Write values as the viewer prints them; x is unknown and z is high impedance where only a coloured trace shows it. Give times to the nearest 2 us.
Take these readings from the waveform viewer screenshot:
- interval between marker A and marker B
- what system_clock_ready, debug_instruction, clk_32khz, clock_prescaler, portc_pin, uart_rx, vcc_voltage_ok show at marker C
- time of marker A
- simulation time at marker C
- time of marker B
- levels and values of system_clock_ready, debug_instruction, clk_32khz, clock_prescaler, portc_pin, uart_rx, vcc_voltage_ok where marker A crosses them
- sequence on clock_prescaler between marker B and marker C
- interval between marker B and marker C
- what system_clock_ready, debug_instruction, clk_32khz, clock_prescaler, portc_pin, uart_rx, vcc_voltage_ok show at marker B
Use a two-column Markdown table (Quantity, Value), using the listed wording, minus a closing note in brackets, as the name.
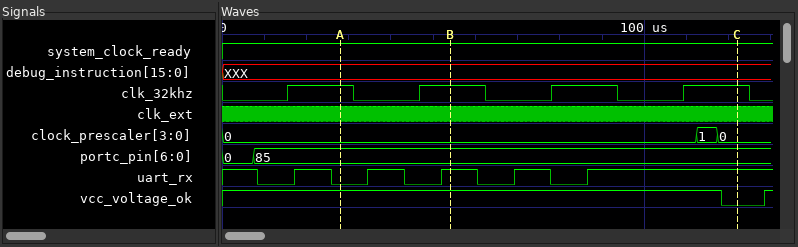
| Quantity | Value |
|---|---|
| interval between marker A and marker B | 26 us |
| what system_clock_ready, debug_instruction, clk_32khz, clock_prescaler, portc_pin, uart_rx, vcc_voltage_ok show at marker C | system_clock_ready=1, debug_instruction=XXX, clk_32khz=1, clock_prescaler=0, portc_pin=85, uart_rx=1, vcc_voltage_ok=0 |
| time of marker A | 28 us |
| simulation time at marker C | 122 us |
| time of marker B | 54 us |
| levels and values of system_clock_ready, debug_instruction, clk_32khz, clock_prescaler, portc_pin, uart_rx, vcc_voltage_ok where marker A crosses them | system_clock_ready=1, debug_instruction=XXX, clk_32khz=1, clock_prescaler=0, portc_pin=85, uart_rx=0, vcc_voltage_ok=1 |
| sequence on clock_prescaler between marker B and marker C | 0, 1, 0 |
| interval between marker B and marker C | 68 us |
| what system_clock_ready, debug_instruction, clk_32khz, clock_prescaler, portc_pin, uart_rx, vcc_voltage_ok show at marker B | system_clock_ready=1, debug_instruction=XXX, clk_32khz=1, clock_prescaler=0, portc_pin=85, uart_rx=1, vcc_voltage_ok=1 |
